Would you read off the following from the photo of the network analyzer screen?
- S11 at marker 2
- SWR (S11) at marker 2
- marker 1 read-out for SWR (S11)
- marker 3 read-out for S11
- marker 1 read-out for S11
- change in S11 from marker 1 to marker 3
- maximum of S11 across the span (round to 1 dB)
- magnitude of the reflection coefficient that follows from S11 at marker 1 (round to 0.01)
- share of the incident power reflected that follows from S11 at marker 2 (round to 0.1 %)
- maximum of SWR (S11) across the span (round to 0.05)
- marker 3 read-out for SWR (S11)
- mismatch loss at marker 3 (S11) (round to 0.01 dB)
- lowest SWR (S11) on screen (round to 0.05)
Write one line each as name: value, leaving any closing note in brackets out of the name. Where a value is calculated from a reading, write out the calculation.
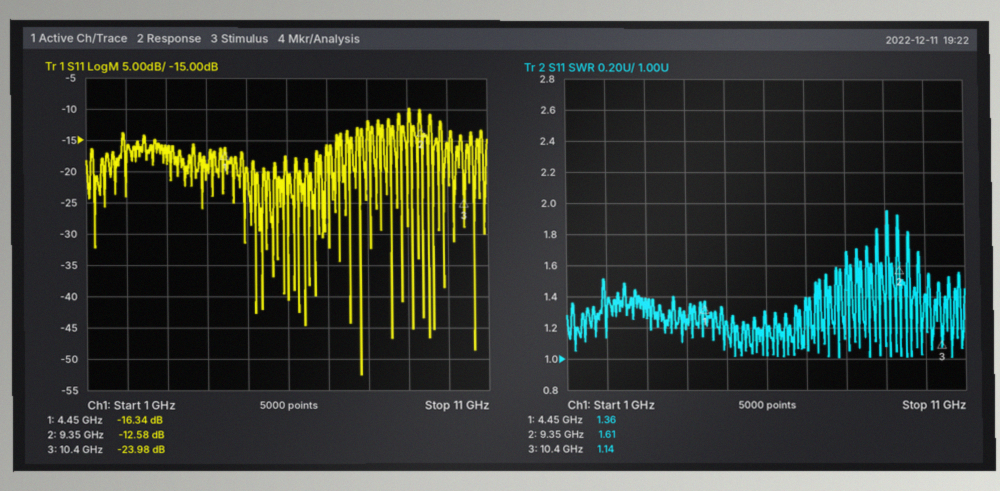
S11 at marker 2: -12.58 dB
SWR (S11) at marker 2: 1.61
marker 1 read-out for SWR: 1.36
marker 3 read-out for S11: -23.98 dB
marker 1 read-out for S11: -16.34 dB
change in S11 from marker 1 to marker 3: -23.98 − (-16.34) = -7.64 dB
maximum of S11 across the span: -10 dB
magnitude of the reflection coefficient that follows from S11 at marker 1: 10^(-16.34/20) ≈ 0.15
share of the incident power reflected that follows from S11 at marker 2: 10^(-12.58/10) ≈ 5.5 %
maximum of SWR (S11) across the span: 1.95
marker 3 read-out for SWR: 1.14
mismatch loss at marker 3 (S11): −10 log10(1 − 10^(-23.98/10)) ≈ 0.02 dB
lowest SWR (S11) on screen: 1.00
